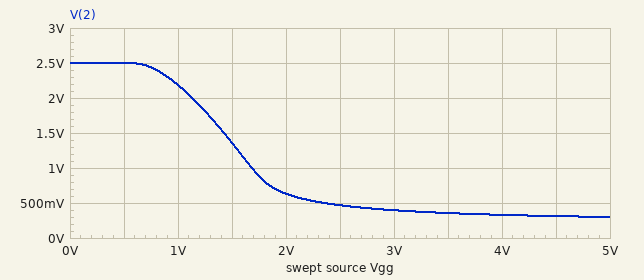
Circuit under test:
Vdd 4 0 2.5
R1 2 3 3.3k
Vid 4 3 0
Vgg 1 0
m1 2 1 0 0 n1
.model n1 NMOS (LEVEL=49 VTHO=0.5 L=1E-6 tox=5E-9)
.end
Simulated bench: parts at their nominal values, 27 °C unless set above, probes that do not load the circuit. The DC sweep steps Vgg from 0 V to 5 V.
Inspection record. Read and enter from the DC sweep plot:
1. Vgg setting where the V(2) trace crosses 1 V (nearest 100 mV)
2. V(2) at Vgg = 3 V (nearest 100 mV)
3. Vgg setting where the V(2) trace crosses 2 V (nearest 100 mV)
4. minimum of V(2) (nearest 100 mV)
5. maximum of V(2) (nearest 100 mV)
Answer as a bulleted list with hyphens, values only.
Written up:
- 1.7 V
- 400 mV
- 1.1 V
- 300 mV
- 2.5 V
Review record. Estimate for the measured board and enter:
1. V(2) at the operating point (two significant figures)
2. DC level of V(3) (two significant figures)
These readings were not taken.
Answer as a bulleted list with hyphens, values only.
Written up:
- 2.5 V
- 2.5 V
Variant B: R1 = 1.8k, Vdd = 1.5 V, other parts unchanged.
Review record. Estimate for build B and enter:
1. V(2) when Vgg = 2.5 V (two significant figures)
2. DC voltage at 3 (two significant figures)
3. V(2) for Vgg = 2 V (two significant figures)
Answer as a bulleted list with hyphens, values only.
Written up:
- 440 mV
- 1.5 V
- 550 mV
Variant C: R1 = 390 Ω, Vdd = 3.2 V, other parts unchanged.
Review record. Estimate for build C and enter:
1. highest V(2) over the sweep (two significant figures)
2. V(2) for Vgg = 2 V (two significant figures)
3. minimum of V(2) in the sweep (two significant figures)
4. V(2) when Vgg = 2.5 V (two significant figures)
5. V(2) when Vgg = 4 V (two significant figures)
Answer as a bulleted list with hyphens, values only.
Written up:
- 3.2 V
- 2.9 V
- 2.1 V
- 2.8 V
- 2.3 V
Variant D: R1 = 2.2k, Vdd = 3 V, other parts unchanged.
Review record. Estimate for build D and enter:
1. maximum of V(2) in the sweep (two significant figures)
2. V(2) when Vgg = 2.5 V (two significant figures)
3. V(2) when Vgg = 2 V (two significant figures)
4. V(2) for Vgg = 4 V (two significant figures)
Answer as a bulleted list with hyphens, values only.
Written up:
- 3.0 V
- 930 mV
- 1.5 V
- 600 mV
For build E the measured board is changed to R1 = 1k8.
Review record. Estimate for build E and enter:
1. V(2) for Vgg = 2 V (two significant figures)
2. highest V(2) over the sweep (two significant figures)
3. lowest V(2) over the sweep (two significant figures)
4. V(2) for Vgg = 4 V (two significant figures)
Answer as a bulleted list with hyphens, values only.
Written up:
- 1.3 V
- 2.5 V
- 520 mV
- 580 mV
